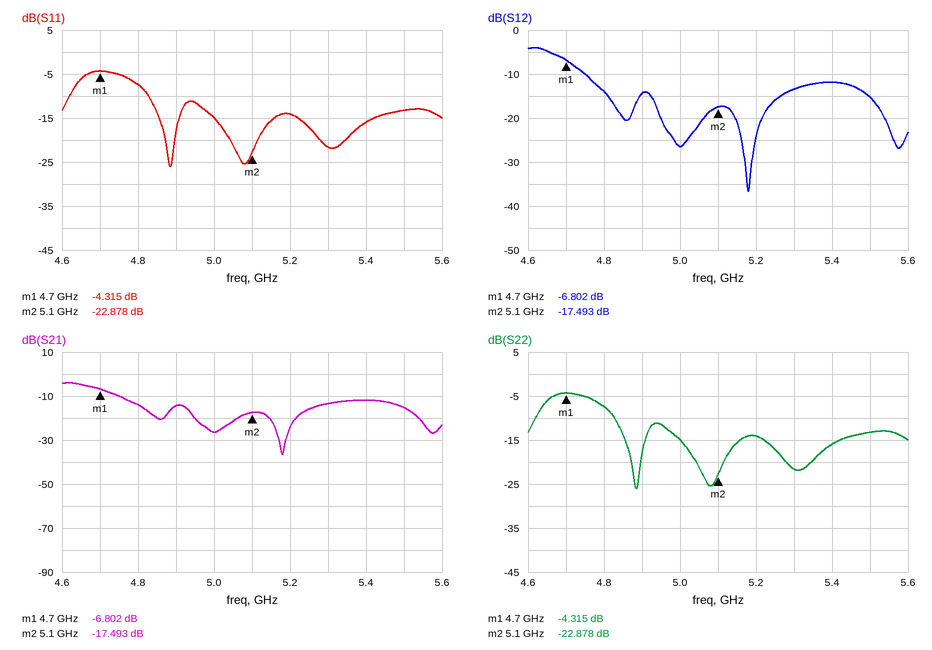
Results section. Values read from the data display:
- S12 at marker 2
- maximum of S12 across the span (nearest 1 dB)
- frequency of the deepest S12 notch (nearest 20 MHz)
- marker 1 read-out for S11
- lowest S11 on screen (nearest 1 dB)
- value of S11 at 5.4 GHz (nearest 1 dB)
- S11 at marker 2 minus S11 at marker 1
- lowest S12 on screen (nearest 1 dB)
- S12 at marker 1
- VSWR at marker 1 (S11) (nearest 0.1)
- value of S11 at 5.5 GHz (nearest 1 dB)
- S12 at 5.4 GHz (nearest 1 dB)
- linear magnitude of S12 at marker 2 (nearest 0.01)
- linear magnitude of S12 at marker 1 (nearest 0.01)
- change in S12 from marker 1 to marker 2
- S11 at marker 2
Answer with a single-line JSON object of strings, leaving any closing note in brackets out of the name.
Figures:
{"S12 at marker 2": "-17.493 dB", "maximum of S12 across the span": "-4 dB", "frequency of the deepest S12 notch": "5.18 GHz", "marker 1 read-out for S11": "-4.315 dB", "lowest S11 on screen": "-26 dB", "value of S11 at 5.4 GHz": "-16 dB", "S11 at marker 2 minus S11 at marker 1": "-18.563 dB", "lowest S12 on screen": "-37 dB", "S12 at marker 1": "-6.802 dB", "VSWR at marker 1 (S11)": "4.1", "value of S11 at 5.5 GHz": "-13 dB", "S12 at 5.4 GHz": "-12 dB", "linear magnitude of S12 at marker 2": "0.13", "linear magnitude of S12 at marker 1": "0.46", "change in S12 from marker 1 to marker 2": "-10.691 dB", "S11 at marker 2": "-22.878 dB"}
